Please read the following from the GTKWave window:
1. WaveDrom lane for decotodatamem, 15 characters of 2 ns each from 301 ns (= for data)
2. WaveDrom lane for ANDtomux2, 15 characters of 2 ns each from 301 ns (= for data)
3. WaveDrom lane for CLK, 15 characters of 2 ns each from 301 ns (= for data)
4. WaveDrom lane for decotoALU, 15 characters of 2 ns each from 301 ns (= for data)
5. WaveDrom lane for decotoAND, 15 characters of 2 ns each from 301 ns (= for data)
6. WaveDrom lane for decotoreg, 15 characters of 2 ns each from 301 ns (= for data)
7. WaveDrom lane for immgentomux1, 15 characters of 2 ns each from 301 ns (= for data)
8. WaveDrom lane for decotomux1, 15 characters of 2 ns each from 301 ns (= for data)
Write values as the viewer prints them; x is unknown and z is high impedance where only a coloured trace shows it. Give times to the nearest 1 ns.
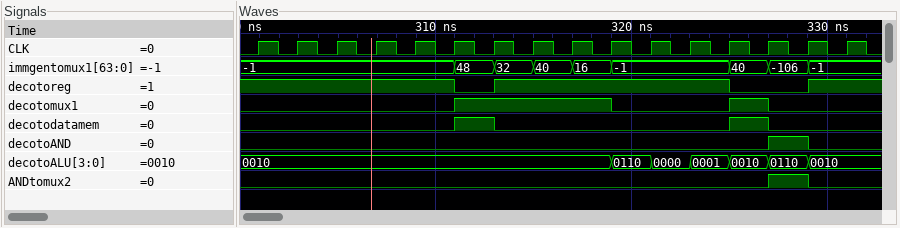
{name: 'decotodatamem', wave: '0....10.....10.'}
{name: 'ANDtomux2', wave: '0............10'}
{name: 'CLK', wave: 'p..............'}
{name: 'decotoALU', wave: '=........======', data: '0010 0110 0000 0001 0010 0110 0010'}
{name: 'decotoAND', wave: '0............10'}
{name: 'decotoreg', wave: '1....01.....0.1'}
{name: 'immgentomux1', wave: '=....=====..===', data: '-1 48 32 40 16 -1 40 -106 -1'}
{name: 'decotomux1', wave: '0....1...0..10.'}
